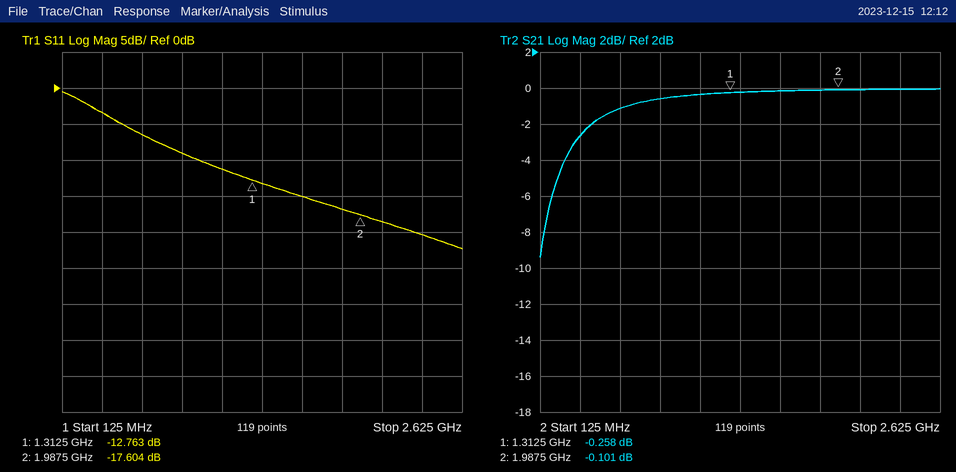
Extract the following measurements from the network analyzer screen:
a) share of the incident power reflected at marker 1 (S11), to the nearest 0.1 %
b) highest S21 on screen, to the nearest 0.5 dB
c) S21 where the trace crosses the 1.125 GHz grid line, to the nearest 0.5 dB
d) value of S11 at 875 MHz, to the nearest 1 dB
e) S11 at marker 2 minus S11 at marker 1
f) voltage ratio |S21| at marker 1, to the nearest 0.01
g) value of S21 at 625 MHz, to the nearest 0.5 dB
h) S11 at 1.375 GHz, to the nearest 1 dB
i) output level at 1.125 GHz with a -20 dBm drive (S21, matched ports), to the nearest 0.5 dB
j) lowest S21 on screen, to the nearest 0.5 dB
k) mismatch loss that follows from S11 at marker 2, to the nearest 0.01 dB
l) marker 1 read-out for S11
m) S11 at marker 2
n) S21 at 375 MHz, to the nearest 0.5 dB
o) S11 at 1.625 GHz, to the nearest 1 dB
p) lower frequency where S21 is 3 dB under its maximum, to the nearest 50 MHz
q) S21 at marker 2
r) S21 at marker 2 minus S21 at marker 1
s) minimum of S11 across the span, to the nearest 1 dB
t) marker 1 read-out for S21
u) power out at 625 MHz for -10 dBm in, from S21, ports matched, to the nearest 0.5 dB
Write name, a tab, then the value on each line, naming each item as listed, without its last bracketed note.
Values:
share of the incident power reflected at marker 1 (S11), to the nearest 0.1 %	5.3 %
highest S21 on screen, to the nearest 0.5 dB	0.0 dB
S21 where the trace crosses the 1.125 GHz grid line, to the nearest 0.5 dB	-0.5 dB
value of S11 at 875 MHz, to the nearest 1 dB	-9 dB
S11 at marker 2 minus S11 at marker 1	-4.841 dB
voltage ratio |S21| at marker 1, to the nearest 0.01	0.97
value of S21 at 625 MHz, to the nearest 0.5 dB	-1.0 dB
S11 at 1.375 GHz, to the nearest 1 dB	-13 dB
output level at 1.125 GHz with a -20 dBm drive (S21, matched ports), to the nearest 0.5 dB	-20.5 dBm
lowest S21 on screen, to the nearest 0.5 dB	-9.5 dB
mismatch loss that follows from S11 at marker 2, to the nearest 0.01 dB	0.08 dB
marker 1 read-out for S11	-12.763 dB
S11 at marker 2	-17.604 dB
S21 at 375 MHz, to the nearest 0.5 dB	-2.5 dB
S11 at 1.625 GHz, to the nearest 1 dB	-15 dB
lower frequency where S21 is 3 dB under its maximum, to the nearest 50 MHz	350 MHz
S21 at marker 2	-0.101 dB
S21 at marker 2 minus S21 at marker 1	0.157 dB
minimum of S11 across the span, to the nearest 1 dB	-22 dB
marker 1 read-out for S21	-0.258 dB
power out at 625 MHz for -10 dBm in, from S21, ports matched, to the nearest 0.5 dB	-11.0 dBm
